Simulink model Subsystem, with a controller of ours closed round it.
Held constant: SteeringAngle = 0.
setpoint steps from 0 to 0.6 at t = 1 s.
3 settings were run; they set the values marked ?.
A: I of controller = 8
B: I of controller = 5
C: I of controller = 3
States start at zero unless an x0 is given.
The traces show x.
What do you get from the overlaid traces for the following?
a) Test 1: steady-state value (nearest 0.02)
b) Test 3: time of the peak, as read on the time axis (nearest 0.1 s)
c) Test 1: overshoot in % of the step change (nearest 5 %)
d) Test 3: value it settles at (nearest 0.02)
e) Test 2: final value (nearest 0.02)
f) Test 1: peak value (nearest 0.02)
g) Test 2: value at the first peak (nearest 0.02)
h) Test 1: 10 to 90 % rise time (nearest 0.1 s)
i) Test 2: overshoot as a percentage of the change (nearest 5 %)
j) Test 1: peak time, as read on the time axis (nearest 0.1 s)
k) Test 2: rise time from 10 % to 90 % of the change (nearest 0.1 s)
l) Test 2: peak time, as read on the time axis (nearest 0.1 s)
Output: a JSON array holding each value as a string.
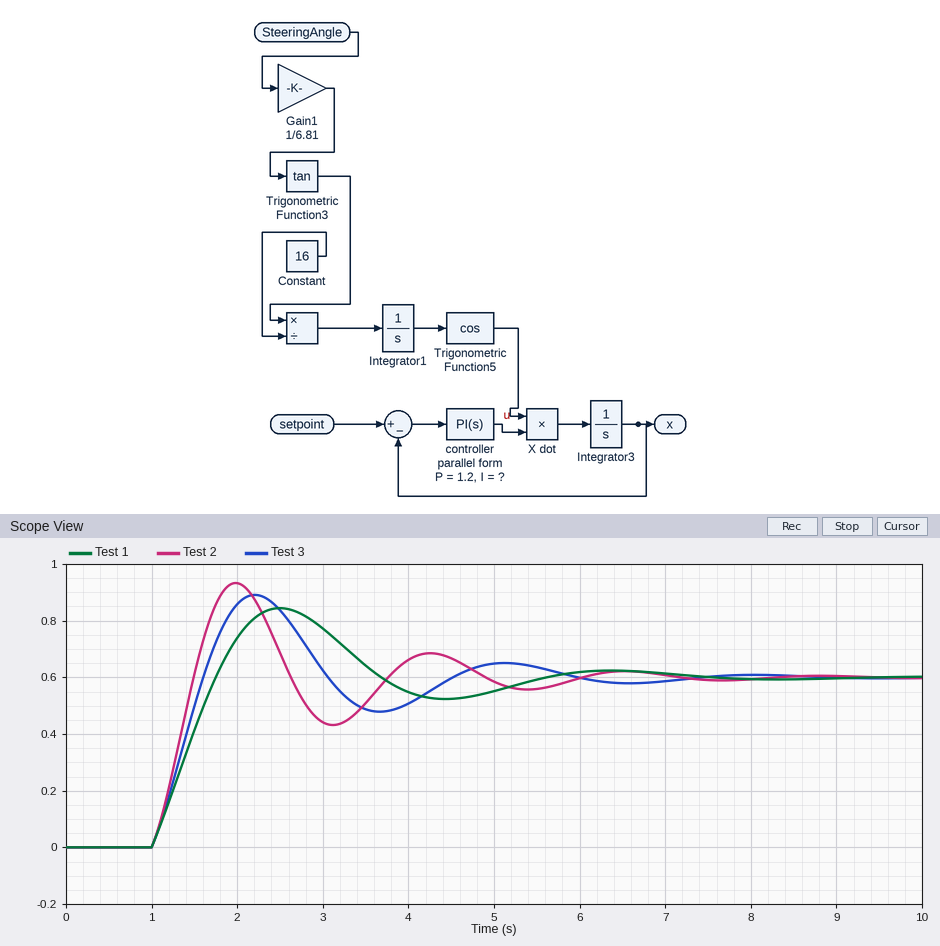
["0.60", "2.2 s", "40 %", "0.60", "0.60", "0.84", "0.94", "0.6 s", "55 %", "2.5 s", "0.4 s", "2.0 s"]
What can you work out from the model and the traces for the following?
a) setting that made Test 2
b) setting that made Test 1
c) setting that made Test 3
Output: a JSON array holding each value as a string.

["A", "C", "B"]
